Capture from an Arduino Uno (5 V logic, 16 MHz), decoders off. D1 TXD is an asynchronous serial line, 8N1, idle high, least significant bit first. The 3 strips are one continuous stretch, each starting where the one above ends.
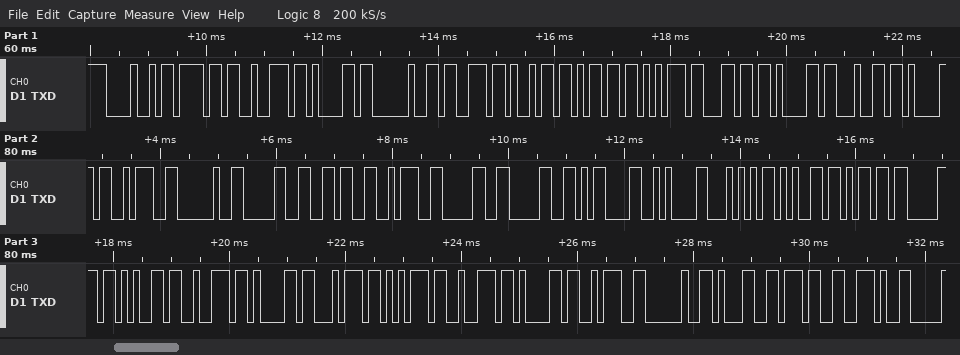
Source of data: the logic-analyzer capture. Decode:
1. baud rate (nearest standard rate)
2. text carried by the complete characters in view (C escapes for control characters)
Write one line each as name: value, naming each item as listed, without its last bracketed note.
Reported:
baud rate: 9600 baud
text carried by the complete characters in view: "Hora simulada: 06:00\r\nTemperatura: 17."
